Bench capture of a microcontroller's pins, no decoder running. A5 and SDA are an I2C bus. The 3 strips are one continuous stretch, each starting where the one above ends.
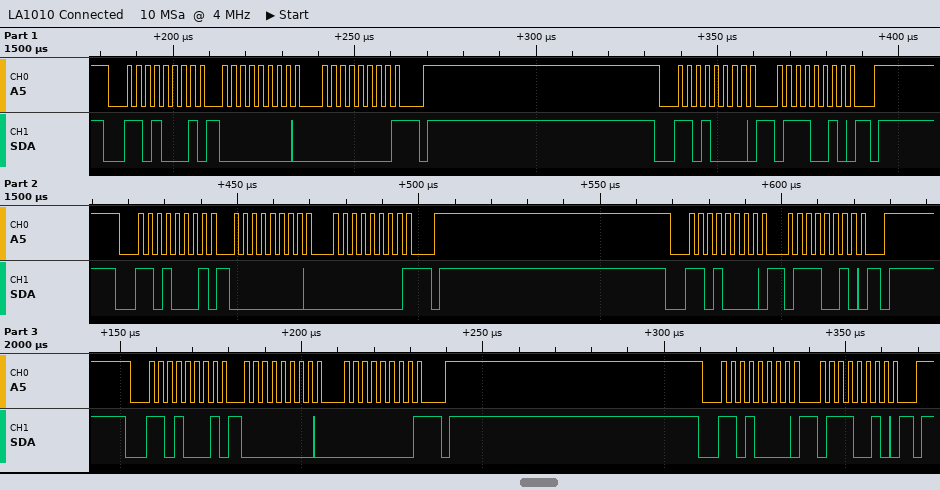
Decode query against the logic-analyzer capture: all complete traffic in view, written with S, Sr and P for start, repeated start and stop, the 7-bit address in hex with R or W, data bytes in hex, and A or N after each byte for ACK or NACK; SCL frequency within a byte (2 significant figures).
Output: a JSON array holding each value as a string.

["S 68R A 00 A 00 N P S 68W A 72 A P S 68R A 00 A 00 N P S 68W A 72 A P S 68R A 00 A 00 N P S 68W A 72 A P", "400 kHz"]
